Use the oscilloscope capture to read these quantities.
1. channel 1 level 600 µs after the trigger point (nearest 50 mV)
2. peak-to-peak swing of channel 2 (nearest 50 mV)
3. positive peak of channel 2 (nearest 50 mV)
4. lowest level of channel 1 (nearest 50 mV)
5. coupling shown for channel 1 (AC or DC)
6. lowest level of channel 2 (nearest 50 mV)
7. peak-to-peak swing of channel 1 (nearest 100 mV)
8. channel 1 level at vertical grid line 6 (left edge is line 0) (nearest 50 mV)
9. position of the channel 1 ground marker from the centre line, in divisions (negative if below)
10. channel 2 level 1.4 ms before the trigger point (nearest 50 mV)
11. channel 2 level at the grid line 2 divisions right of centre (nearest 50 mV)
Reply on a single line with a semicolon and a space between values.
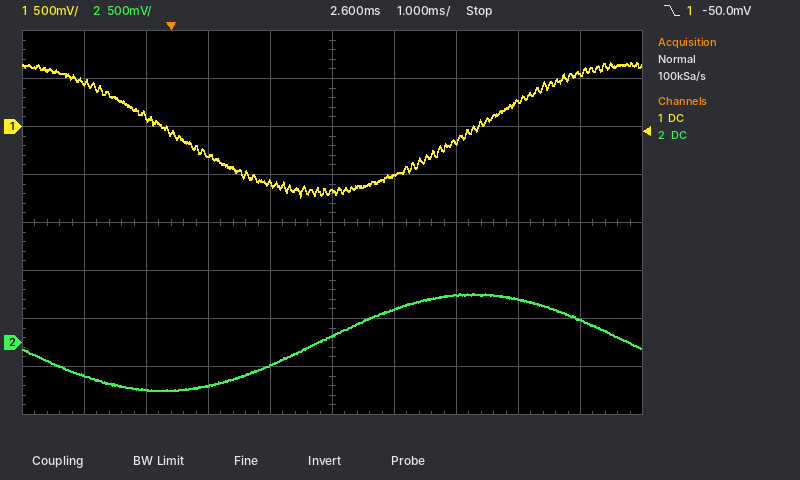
-300 mV; 1.00 V; 500 mV; -750 mV; DC; -500 mV; 1.40 V; -500 mV; +2.0 div; -350 mV; 500 mV
